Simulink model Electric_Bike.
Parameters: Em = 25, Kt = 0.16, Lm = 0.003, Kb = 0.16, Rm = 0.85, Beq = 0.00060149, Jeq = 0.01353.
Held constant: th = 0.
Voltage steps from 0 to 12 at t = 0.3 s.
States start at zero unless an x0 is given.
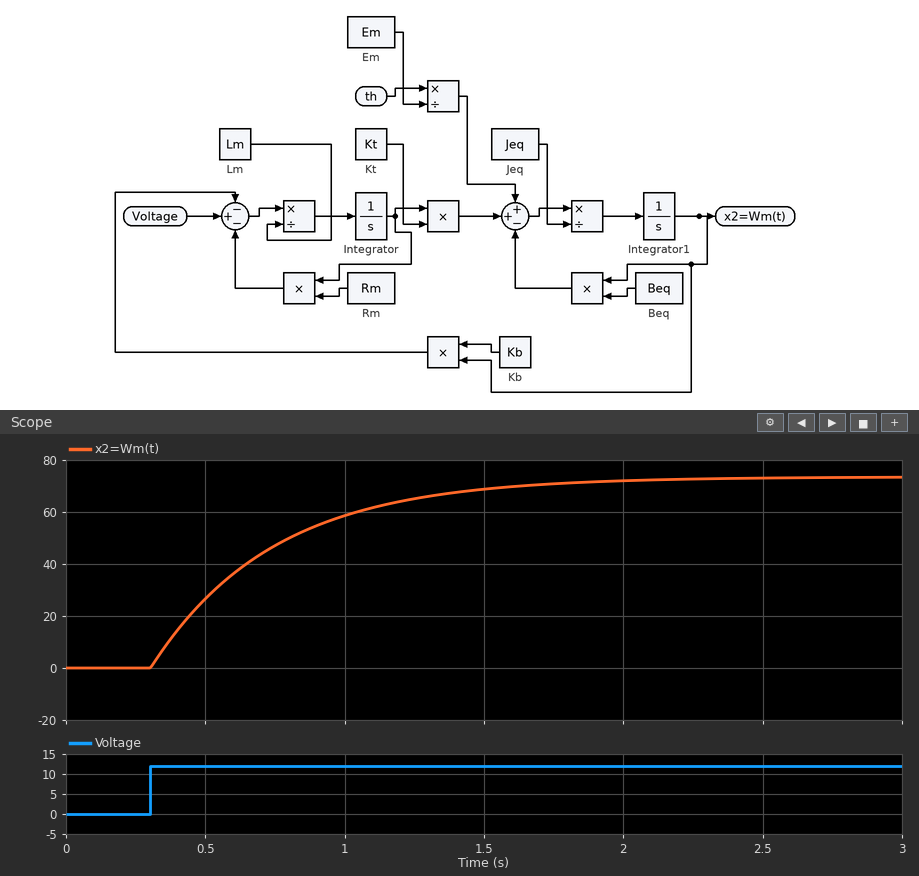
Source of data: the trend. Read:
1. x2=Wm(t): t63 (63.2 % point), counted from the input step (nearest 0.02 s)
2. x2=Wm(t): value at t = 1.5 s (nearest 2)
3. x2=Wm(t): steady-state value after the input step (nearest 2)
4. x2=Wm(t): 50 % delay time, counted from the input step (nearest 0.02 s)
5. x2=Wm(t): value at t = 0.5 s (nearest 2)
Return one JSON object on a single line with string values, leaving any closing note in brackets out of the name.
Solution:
{"x2=Wm(t): t63 (63.2 % point), counted from the input step": "0.44 s", "x2=Wm(t): value at t = 1.5 s": "68", "x2=Wm(t): steady-state value after the input step": "74", "x2=Wm(t): 50 % delay time, counted from the input step": "0.30 s", "x2=Wm(t): value at t = 0.5 s": "26"}
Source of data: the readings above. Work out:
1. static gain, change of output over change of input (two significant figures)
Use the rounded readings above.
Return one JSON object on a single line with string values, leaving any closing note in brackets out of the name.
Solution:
{"static gain, change of output over change of input": "6.2"}
